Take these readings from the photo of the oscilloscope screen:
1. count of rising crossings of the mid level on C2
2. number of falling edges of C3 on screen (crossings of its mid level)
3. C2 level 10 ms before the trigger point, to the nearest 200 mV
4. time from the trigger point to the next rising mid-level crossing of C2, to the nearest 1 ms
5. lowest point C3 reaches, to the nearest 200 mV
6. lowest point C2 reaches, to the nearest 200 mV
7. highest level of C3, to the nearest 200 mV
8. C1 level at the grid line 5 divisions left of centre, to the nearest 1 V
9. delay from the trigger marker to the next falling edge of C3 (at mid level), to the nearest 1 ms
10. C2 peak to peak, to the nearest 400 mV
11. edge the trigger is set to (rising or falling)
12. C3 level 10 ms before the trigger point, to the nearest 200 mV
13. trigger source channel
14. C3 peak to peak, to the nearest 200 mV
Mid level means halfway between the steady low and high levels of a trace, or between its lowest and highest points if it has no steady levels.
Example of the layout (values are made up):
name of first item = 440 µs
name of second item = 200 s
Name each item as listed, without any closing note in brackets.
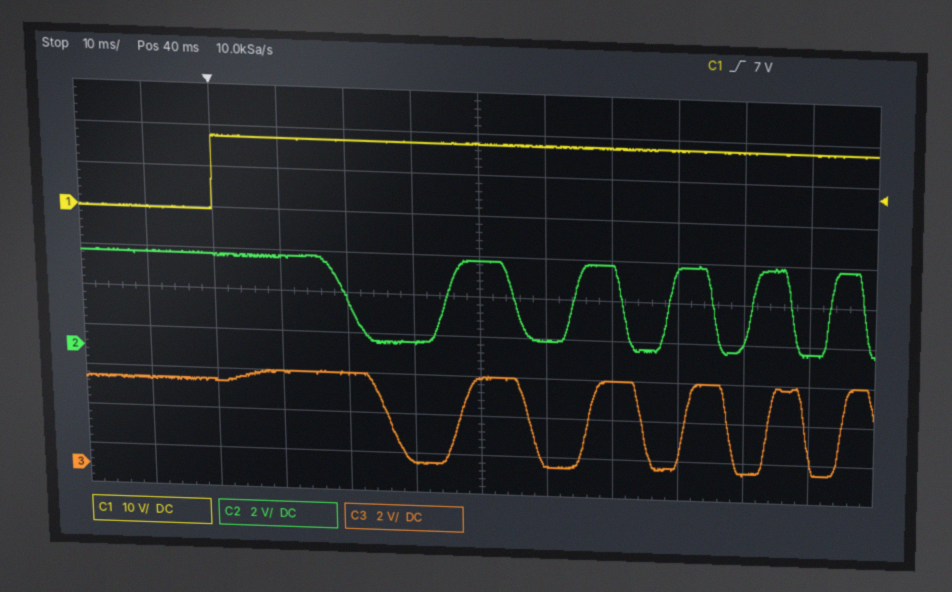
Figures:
count of rising crossings of the mid level on C2 = 5
number of falling edges of C3 on screen = 5
C2 level 10 ms before the trigger point, to the nearest 200 mV = 4.8 V
time from the trigger point to the next rising mid-level crossing of C2, to the nearest 1 ms = 35 ms
lowest point C3 reaches, to the nearest 200 mV = 400 mV
lowest point C2 reaches, to the nearest 200 mV = 600 mV
highest level of C3, to the nearest 200 mV = 5.0 V
C1 level at the grid line 5 divisions left of centre, to the nearest 1 V = 0 V
delay from the trigger marker to the next falling edge of C3 (at mid level), to the nearest 1 ms = 26 ms
C2 peak to peak, to the nearest 400 mV = 4.4 V
edge the trigger is set to = rising
C3 level 10 ms before the trigger point, to the nearest 200 mV = 4.4 V
trigger source channel = C1
C3 peak to peak, to the nearest 200 mV = 4.6 V
